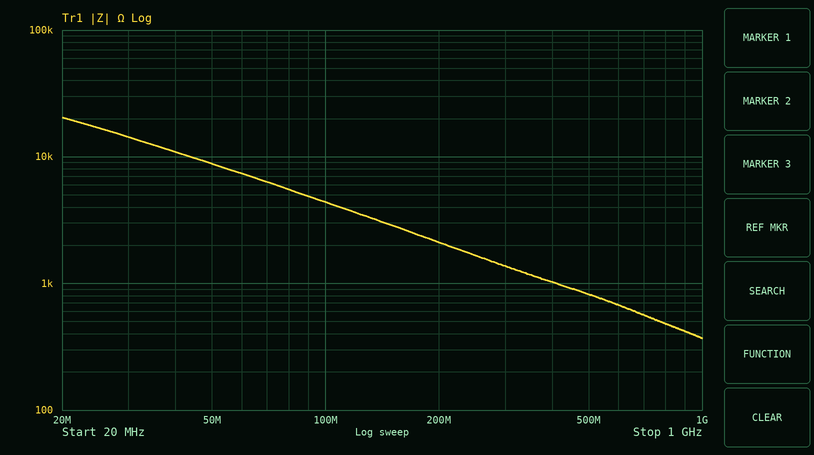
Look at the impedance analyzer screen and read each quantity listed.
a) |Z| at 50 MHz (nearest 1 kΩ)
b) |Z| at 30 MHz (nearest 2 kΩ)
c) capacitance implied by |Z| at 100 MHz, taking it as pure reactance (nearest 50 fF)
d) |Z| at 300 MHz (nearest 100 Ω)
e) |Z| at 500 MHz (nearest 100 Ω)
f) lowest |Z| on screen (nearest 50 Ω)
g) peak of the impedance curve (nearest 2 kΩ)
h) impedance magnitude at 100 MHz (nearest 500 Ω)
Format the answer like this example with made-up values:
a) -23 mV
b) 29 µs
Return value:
a) 9 kΩ
b) 14 kΩ
c) 350 fF
d) 1.4 kΩ
e) 800 Ω
f) 350 Ω
g) 20 kΩ
h) 4.5 kΩ
